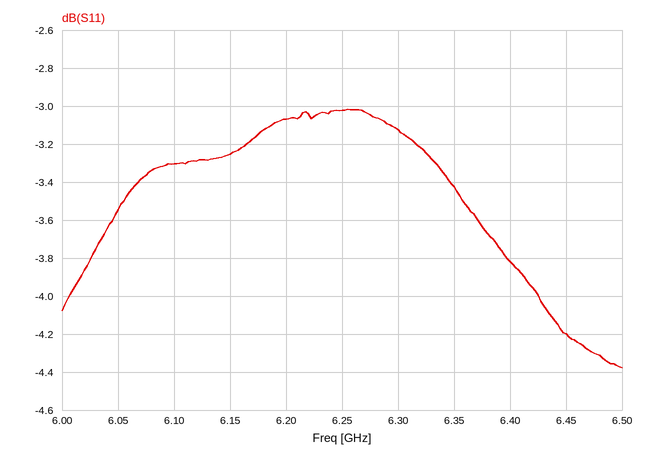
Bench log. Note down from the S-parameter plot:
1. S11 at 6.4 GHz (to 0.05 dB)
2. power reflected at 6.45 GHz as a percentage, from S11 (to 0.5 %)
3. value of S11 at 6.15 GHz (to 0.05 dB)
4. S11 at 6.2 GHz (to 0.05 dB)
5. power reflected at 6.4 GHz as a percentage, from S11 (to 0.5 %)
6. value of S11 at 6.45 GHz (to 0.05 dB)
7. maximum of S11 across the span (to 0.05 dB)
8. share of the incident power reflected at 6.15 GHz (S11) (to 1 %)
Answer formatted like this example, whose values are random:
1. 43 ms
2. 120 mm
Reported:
1. -3.80 dB
2. 38.0 %
3. -3.25 dB
4. -3.05 dB
5. 41.5 %
6. -4.20 dB
7. -3.00 dB
8. 47 %
